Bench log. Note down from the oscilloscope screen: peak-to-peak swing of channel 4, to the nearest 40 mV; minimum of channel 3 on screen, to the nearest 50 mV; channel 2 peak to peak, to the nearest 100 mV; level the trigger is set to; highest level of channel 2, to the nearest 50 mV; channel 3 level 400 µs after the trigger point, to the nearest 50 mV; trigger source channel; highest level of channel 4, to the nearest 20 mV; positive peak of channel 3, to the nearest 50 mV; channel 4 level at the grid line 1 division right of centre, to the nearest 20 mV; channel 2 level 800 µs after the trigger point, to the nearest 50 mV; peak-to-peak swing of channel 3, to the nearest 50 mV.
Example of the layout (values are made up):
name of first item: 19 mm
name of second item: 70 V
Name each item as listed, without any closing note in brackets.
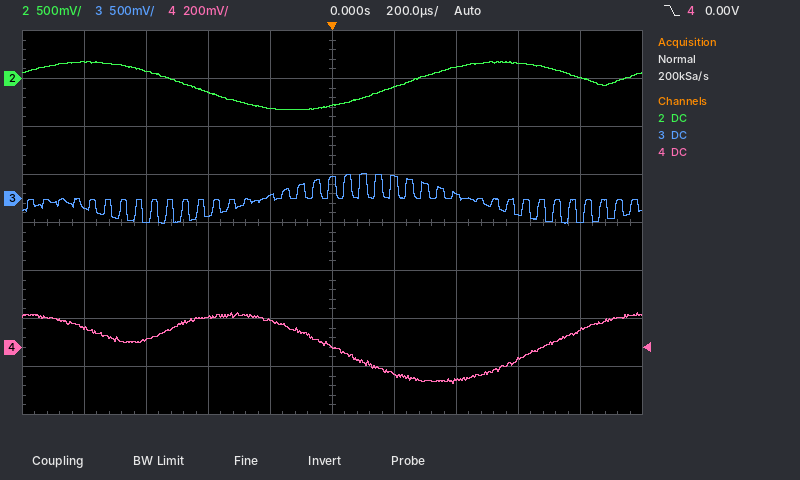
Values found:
peak-to-peak swing of channel 4, to the nearest 40 mV: 280 mV
minimum of channel 3 on screen, to the nearest 50 mV: -250 mV
channel 2 peak to peak, to the nearest 100 mV: 500 mV
level the trigger is set to: 0.00 V
highest level of channel 2, to the nearest 50 mV: 200 mV
channel 3 level 400 µs after the trigger point, to the nearest 50 mV: 50 mV
trigger source channel: channel 4
highest level of channel 4, to the nearest 20 mV: 140 mV
positive peak of channel 3, to the nearest 50 mV: 250 mV
channel 4 level at the grid line 1 division right of centre, to the nearest 20 mV: -120 mV
channel 2 level 800 µs after the trigger point, to the nearest 50 mV: 0 mV
peak-to-peak swing of channel 3, to the nearest 50 mV: 500 mV
